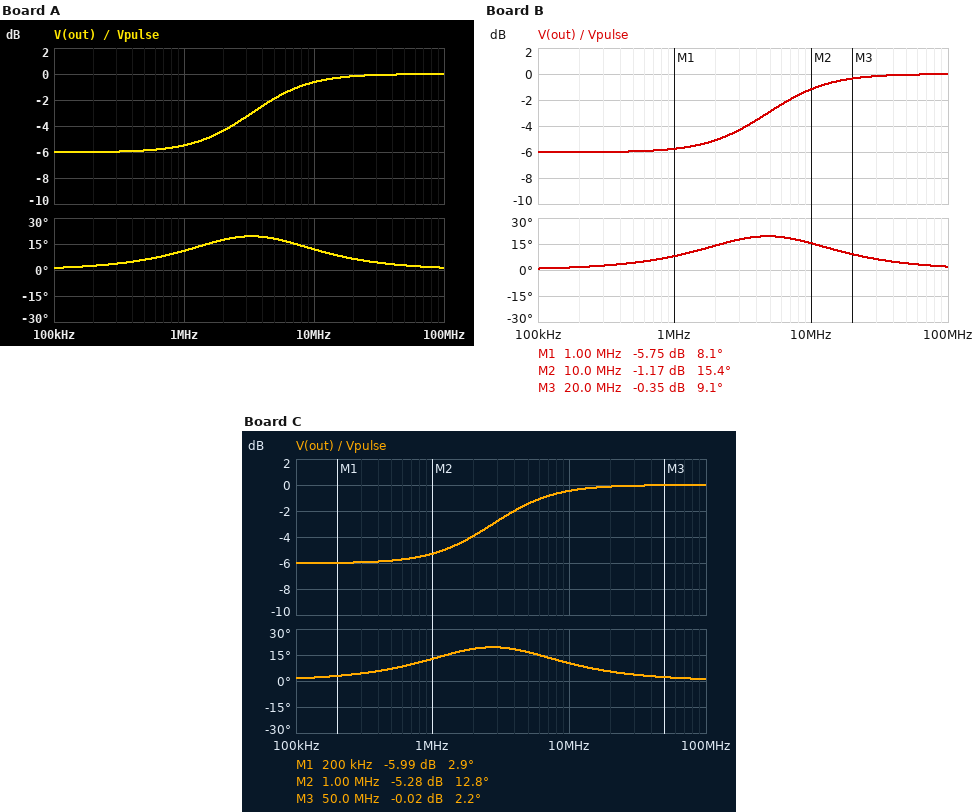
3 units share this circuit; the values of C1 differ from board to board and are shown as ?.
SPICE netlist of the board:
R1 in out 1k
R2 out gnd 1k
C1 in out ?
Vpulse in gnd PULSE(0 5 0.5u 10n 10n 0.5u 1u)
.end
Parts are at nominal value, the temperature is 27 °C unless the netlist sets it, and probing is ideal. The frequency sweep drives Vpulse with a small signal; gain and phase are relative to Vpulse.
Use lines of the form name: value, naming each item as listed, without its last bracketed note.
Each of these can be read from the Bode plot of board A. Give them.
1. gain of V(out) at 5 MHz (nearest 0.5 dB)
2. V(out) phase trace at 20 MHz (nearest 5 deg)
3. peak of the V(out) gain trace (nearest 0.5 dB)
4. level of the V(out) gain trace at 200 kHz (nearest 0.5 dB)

gain of V(out) at 5 MHz: -2.0 dB
V(out) phase trace at 20 MHz: 5 deg
peak of the V(out) gain trace: 0 dB
level of the V(out) gain trace at 200 kHz: -6.0 dB
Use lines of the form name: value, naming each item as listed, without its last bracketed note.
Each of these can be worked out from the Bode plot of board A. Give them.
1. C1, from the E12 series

C1, from the E12 series: 68 pF
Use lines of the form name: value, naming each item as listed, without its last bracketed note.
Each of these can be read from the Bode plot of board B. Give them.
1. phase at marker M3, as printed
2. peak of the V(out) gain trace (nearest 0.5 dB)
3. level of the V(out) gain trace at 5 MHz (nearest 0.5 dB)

phase at marker M3, as printed: 9.1 deg
peak of the V(out) gain trace: 0 dB
level of the V(out) gain trace at 5 MHz: -3.0 dB
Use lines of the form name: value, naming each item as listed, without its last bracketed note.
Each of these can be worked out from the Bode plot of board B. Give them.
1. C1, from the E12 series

C1, from the E12 series: 47 pF
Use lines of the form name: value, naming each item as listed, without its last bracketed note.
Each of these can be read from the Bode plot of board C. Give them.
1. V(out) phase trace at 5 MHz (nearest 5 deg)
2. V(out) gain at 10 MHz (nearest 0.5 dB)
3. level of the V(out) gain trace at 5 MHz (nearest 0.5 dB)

V(out) phase trace at 5 MHz: 15 deg
V(out) gain at 10 MHz: -0.5 dB
level of the V(out) gain trace at 5 MHz: -1.5 dB
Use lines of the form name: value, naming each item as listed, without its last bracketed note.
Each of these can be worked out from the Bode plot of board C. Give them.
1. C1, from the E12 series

C1, from the E12 series: 82 pF
